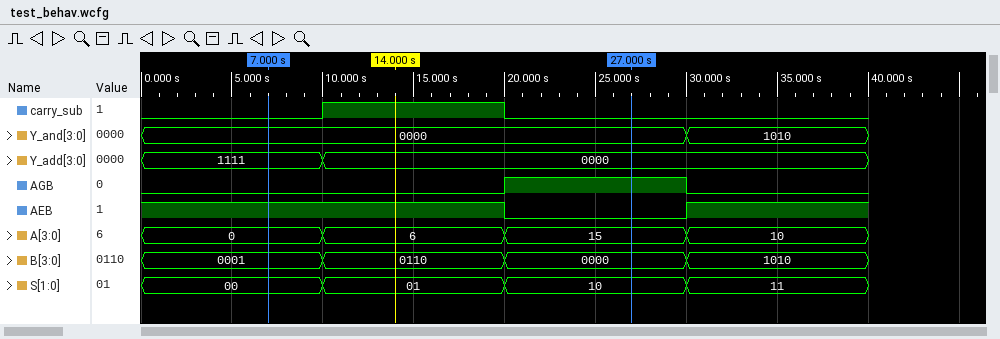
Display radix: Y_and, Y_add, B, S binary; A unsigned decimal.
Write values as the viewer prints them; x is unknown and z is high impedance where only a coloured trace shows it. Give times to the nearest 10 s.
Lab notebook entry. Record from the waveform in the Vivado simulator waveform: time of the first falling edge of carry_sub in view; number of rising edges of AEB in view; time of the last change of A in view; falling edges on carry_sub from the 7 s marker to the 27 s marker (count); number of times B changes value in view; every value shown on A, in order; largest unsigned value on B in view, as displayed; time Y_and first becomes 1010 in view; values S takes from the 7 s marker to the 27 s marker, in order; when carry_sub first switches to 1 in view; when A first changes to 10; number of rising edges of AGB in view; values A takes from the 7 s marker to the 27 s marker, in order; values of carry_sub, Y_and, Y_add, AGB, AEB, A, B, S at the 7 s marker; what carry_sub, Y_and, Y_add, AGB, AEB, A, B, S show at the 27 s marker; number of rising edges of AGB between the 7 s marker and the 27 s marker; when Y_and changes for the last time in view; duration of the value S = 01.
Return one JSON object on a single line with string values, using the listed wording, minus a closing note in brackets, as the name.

{"time of the first falling edge of carry_sub in view": "20 s", "number of rising edges of AEB in view": "1", "time of the last change of A in view": "30 s", "falling edges on carry_sub from the 7 s marker to the 27 s marker": "1", "number of times B changes value in view": "3", "every value shown on A, in order": "0, 6, 15, 10", "largest unsigned value on B in view, as displayed": "1010", "time Y_and first becomes 1010 in view": "30 s", "values S takes from the 7 s marker to the 27 s marker, in order": "00, 01, 10", "when carry_sub first switches to 1 in view": "10 s", "when A first changes to 10": "30 s", "number of rising edges of AGB in view": "1", "values A takes from the 7 s marker to the 27 s marker, in order": "0, 6, 15", "values of carry_sub, Y_and, Y_add, AGB, AEB, A, B, S at the 7 s marker": "carry_sub=0, Y_and=0000, Y_add=1111, AGB=0, AEB=1, A=0, B=0001, S=00", "what carry_sub, Y_and, Y_add, AGB, AEB, A, B, S show at the 27 s marker": "carry_sub=0, Y_and=0000, Y_add=0000, AGB=1, AEB=0, A=15, B=0000, S=10", "number of rising edges of AGB between the 7 s marker and the 27 s marker": "1", "when Y_and changes for the last time in view": "30 s", "duration of the value S = 01": "10 s"}
